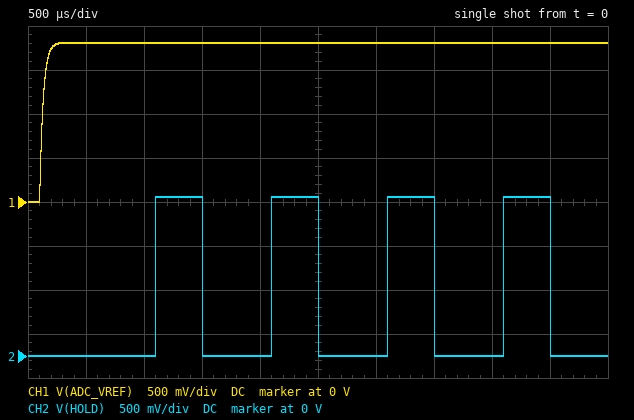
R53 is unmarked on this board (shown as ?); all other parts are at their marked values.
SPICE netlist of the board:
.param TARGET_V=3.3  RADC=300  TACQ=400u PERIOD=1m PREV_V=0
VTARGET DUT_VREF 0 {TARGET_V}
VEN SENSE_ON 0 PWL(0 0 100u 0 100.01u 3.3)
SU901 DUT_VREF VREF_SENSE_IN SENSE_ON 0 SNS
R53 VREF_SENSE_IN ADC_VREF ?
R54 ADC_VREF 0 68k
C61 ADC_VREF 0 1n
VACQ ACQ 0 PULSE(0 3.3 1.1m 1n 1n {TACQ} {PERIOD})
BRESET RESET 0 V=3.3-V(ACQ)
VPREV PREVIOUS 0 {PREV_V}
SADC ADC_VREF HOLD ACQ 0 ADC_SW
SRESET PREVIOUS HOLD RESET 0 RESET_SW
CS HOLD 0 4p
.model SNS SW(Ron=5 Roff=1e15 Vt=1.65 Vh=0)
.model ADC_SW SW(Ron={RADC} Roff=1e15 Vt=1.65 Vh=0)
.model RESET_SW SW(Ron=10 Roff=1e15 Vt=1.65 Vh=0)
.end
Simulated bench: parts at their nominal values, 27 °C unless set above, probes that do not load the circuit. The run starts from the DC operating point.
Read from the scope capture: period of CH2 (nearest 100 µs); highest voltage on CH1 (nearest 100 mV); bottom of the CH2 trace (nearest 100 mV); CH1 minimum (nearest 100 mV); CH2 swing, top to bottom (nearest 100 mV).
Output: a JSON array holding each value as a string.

["1.0 ms", "1.8 V", "0 V", "0 V", "1.8 V"]
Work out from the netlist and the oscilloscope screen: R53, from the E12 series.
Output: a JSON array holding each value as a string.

["56 kΩ"]
